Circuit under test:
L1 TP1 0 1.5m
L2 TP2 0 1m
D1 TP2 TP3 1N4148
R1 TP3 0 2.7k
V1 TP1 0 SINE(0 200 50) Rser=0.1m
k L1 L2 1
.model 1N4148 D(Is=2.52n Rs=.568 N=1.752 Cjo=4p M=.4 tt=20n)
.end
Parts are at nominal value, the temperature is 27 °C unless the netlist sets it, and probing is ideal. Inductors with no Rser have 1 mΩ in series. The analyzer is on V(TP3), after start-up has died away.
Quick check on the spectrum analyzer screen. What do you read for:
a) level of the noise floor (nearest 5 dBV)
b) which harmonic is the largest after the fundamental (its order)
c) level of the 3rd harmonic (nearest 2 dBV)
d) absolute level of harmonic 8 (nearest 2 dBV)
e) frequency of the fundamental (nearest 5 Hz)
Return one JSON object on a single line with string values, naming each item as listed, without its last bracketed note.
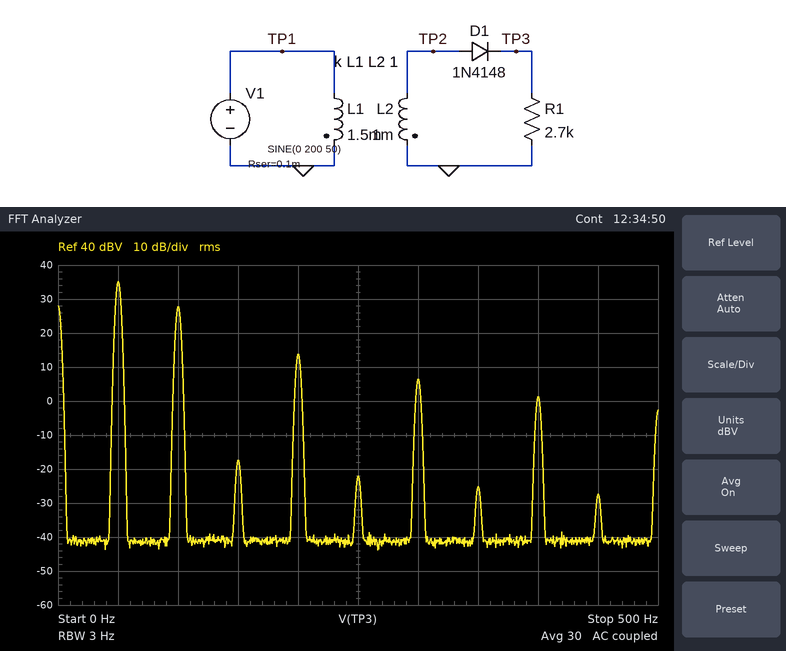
{"level of the noise floor": "-40 dBV", "which harmonic is the largest after the fundamental": "2", "level of the 3rd harmonic": "-18 dBV", "absolute level of harmonic 8": "2 dBV", "frequency of the fundamental": "50 Hz"}
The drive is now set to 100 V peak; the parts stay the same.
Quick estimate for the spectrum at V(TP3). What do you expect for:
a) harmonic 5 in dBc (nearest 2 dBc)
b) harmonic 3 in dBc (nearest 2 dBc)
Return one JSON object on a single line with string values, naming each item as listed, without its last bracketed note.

{"harmonic 5 in dBc": "-52 dBc", "harmonic 3 in dBc": "-48 dBc"}
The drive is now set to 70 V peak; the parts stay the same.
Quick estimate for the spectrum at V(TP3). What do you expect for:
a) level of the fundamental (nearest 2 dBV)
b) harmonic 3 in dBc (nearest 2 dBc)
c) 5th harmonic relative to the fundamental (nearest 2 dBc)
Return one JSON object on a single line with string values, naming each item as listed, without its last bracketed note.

{"level of the fundamental": "26 dBV", "harmonic 3 in dBc": "-46 dBc", "5th harmonic relative to the fundamental": "-50 dBc"}
